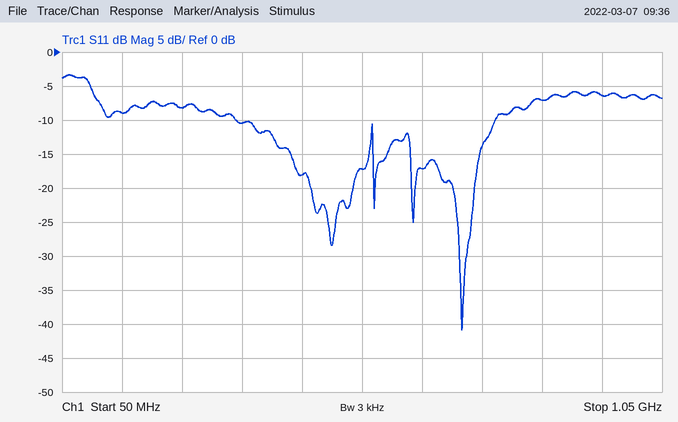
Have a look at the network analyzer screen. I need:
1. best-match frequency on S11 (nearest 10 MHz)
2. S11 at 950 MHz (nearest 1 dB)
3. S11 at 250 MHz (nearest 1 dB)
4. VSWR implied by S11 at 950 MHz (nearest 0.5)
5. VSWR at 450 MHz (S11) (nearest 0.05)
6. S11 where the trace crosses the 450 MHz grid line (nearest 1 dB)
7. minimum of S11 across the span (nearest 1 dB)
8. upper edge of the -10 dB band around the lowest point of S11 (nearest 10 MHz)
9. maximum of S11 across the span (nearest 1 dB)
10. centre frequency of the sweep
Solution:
720 MHz
-6 dB
-8 dB
3.0
1.30
-18 dB
-41 dB
770 MHz
-3 dB
550 MHz
